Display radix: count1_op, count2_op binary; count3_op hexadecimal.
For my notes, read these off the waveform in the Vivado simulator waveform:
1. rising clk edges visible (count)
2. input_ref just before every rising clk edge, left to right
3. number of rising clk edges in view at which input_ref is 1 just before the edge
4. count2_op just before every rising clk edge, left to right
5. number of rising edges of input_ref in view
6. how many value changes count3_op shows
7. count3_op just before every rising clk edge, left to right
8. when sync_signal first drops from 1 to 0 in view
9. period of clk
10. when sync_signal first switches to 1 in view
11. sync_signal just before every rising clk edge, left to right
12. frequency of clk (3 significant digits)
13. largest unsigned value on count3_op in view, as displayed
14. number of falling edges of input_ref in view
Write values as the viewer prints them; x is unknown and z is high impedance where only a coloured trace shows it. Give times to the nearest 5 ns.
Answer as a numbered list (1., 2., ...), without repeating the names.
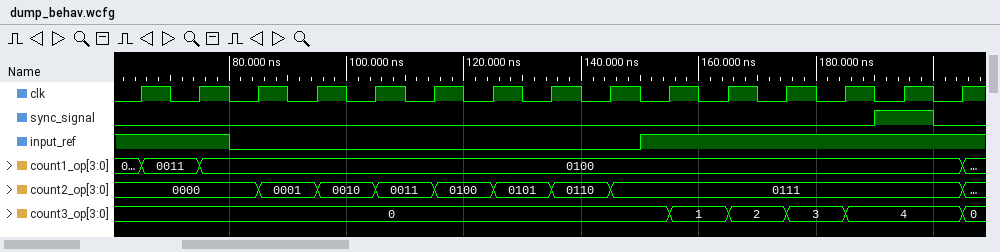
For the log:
1. 15
2. 1 1 0 0 0 0 0 0 0 1 1 1 1 1 1
3. 8
4. 0000, 0000, 0000, 0001, 0010, 0011, 0100, 0101, 0110, 0111, 0111, 0111, 0111, 0111, 0111
5. 1
6. 5
7. 0, 0, 0, 0, 0, 0, 0, 0, 0, 0, 1, 2, 3, 4, 4
8. 200 ns
9. 10 ns
10. 190 ns
11. 0 0 0 0 0 0 0 0 0 0 0 0 0 1 0
12. 100 MHz
13. 4
14. 1
